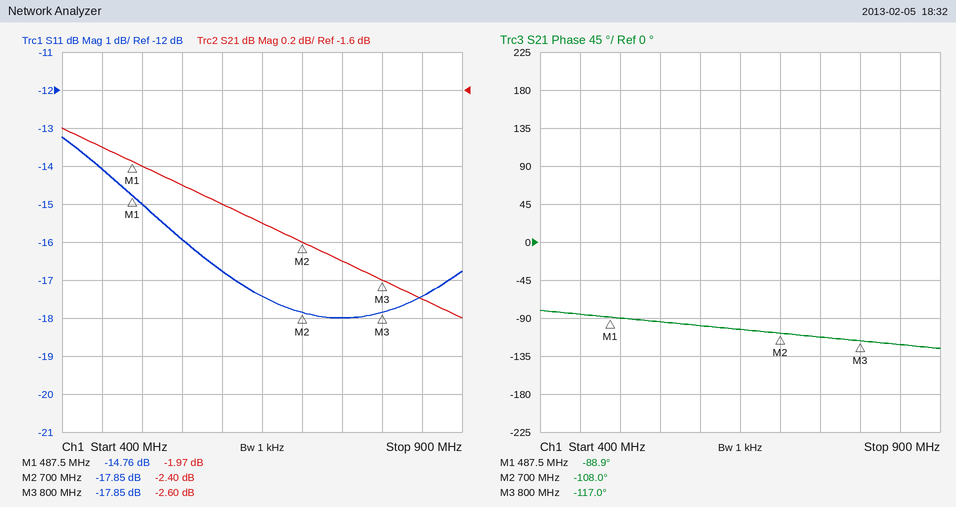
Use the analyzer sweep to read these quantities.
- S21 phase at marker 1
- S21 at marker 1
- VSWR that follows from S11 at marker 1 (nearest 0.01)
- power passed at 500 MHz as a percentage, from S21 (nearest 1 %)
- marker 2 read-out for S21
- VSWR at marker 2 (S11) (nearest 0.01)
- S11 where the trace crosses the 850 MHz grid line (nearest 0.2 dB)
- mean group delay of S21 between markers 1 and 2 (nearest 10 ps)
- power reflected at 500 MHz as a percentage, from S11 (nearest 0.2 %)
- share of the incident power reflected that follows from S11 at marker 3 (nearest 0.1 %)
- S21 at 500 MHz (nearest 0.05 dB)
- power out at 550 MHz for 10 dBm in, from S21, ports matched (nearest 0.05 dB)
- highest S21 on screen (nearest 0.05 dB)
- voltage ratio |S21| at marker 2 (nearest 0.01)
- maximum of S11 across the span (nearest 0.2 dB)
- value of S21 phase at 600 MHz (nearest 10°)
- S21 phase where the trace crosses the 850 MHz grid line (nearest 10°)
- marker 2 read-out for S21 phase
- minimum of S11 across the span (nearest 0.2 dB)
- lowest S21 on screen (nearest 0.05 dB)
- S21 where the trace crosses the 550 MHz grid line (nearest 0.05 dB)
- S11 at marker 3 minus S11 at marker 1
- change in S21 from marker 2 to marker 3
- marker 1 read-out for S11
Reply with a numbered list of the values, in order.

1. -88.9°
2. -1.97 dB
3. 1.45
4. 63 %
5. -2.40 dB
6. 1.29
7. -17.4 dB
8. 250 ps
9. 3.2 %
10. 1.6 %
11. -2.00 dB
12. 7.90 dBm
13. -1.80 dB
14. 0.76
15. -13.2 dB
16. -100°
17. -120°
18. -108.0°
19. -18.0 dB
20. -2.80 dB
21. -2.10 dB
22. -3.09 dB
23. -0.20 dB
24. -14.76 dB
